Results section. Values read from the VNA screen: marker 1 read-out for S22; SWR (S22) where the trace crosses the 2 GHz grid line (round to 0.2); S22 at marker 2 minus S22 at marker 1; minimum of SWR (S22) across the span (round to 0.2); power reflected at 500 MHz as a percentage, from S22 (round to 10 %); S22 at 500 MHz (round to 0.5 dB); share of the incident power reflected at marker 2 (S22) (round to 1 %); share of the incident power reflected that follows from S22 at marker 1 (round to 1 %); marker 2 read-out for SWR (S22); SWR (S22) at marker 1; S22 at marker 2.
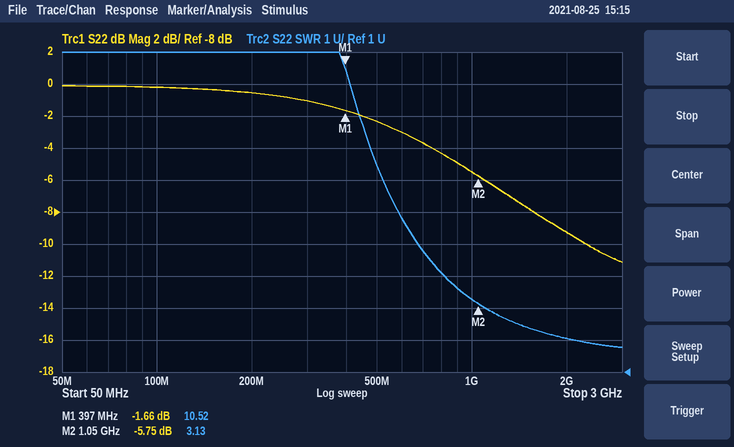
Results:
-1.66 dB
2.0
-4.09 dB
1.8
60 %
-2.5 dB
27 %
68 %
3.13
10.52
-5.75 dB
